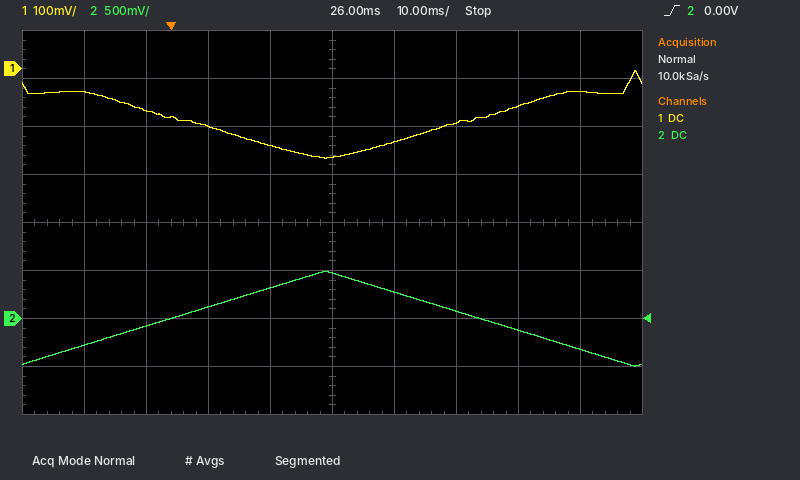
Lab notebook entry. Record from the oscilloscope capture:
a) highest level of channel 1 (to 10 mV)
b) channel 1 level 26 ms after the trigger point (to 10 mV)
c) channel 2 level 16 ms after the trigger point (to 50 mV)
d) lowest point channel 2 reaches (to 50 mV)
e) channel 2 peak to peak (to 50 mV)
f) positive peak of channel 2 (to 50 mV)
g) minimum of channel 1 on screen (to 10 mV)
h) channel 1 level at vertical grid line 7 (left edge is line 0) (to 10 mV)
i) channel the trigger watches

0 mV
-180 mV
300 mV
-500 mV
1.00 V
500 mV
-190 mV
-110 mV
channel 2
